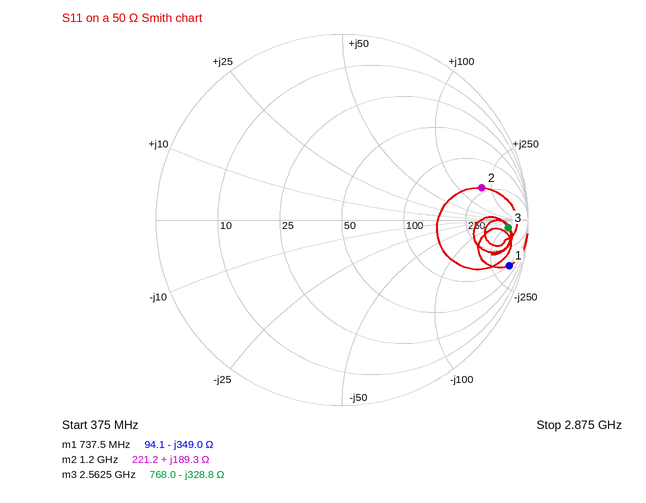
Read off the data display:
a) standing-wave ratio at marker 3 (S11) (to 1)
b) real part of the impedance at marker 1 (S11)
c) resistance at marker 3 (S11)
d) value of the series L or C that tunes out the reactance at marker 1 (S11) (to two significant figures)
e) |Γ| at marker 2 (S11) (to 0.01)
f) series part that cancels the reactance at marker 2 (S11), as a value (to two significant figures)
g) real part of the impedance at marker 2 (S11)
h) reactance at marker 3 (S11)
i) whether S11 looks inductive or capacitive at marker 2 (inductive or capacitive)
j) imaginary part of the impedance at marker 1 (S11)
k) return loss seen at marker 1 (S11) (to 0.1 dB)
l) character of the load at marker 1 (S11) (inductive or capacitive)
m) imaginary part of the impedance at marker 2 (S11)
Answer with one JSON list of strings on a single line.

["18", "94.1 Ω", "768.0 Ω", "75 nH", "0.77", "700 fF", "221.2 Ω", "-328.8 Ω", "inductive", "-349.0 Ω", "0.6 dB", "capacitive", "+189.3 Ω"]
